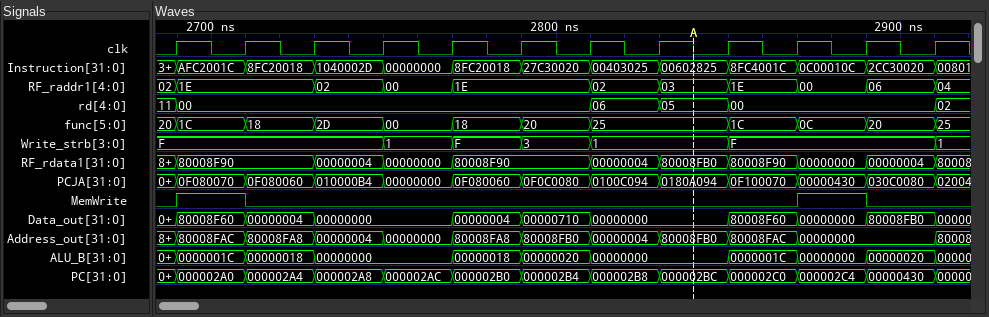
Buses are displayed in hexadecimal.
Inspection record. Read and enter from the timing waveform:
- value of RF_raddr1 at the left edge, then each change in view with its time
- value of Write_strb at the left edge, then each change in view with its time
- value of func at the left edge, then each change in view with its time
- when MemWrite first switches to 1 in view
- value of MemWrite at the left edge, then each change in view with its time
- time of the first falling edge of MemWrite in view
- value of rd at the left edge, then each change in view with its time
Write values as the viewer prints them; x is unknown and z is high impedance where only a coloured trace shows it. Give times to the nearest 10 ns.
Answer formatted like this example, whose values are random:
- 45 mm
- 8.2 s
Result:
- 02, 1E at 2690 ns, 02 at 2730 ns, 00 at 2750 ns, 1E at 2770 ns, 02 at 2810 ns, 03 at 2830 ns, 1E at 2850 ns, 00 at 2870 ns, 06 at 2890 ns, 04 at 2910 ns
- F, 1 at 2750 ns, F at 2770 ns, 3 at 2790 ns, 1 at 2810 ns, F at 2850 ns, 1 at 2910 ns
- 20, 1C at 2690 ns, 18 at 2710 ns, 2D at 2730 ns, 00 at 2750 ns, 18 at 2770 ns, 20 at 2790 ns, 25 at 2810 ns, 1C at 2850 ns, 0C at 2870 ns, 20 at 2890 ns, 25 at 2910 ns
- 2690 ns
- 0, 1 at 2690 ns, 0 at 2710 ns, 1 at 2870 ns, 0 at 2890 ns
- 2710 ns
- 11, 00 at 2690 ns, 06 at 2810 ns, 05 at 2830 ns, 00 at 2850 ns, 02 at 2910 ns
